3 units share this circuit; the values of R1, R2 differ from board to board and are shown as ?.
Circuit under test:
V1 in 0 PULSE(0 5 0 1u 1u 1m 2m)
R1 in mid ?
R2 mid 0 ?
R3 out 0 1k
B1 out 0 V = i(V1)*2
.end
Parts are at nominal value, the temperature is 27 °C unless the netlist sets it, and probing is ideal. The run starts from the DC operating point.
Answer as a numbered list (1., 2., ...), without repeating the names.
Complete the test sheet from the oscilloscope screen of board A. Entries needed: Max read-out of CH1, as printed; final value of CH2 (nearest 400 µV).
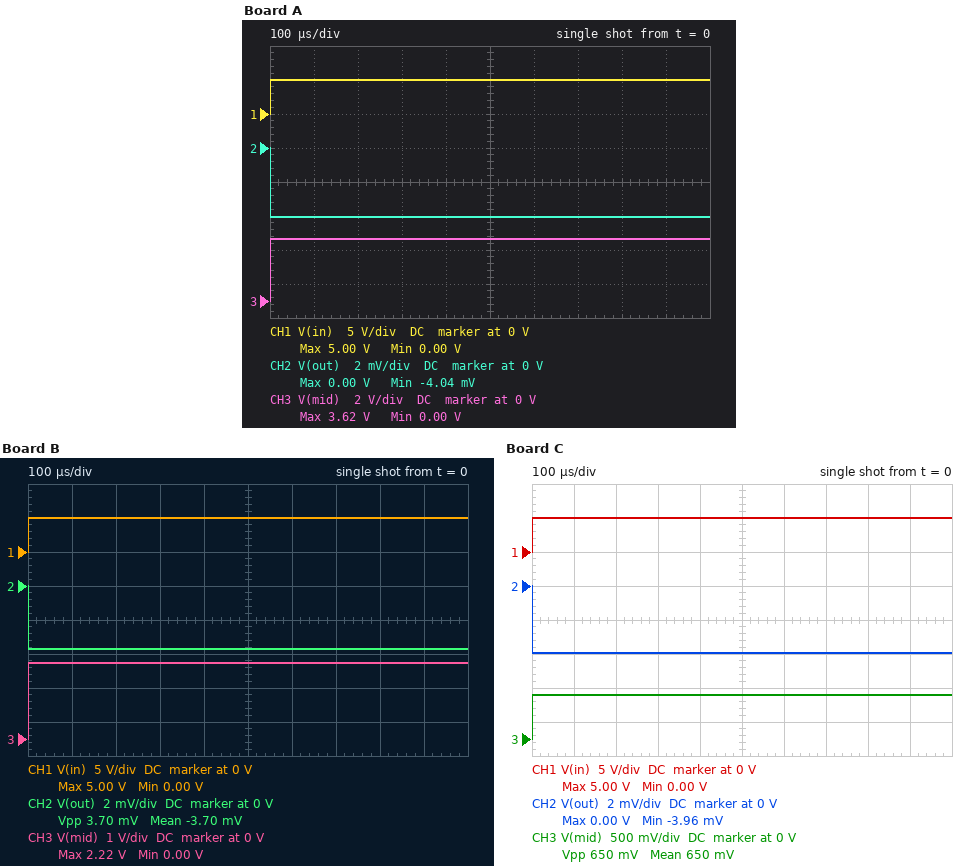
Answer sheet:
1. 5.00 V
2. -4.0 mV
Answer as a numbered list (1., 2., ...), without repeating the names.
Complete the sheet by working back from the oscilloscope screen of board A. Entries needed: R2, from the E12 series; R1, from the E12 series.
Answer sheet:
1. 1.8 kΩ
2. 680 Ω
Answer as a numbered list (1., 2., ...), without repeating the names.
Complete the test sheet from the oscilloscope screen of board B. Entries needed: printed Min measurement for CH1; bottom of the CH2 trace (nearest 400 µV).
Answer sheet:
1. 0.00 V
2. -3.6 mV
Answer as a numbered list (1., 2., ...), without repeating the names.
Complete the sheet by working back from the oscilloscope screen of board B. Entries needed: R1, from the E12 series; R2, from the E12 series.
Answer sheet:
1. 1.5 kΩ
2. 1.2 kΩ
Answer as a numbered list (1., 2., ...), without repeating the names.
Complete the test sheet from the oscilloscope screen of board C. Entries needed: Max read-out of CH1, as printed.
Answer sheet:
1. 5.00 V
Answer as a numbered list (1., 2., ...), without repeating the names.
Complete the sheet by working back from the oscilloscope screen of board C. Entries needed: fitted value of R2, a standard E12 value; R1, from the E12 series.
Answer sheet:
1. 330 Ω
2. 2.2 kΩ
